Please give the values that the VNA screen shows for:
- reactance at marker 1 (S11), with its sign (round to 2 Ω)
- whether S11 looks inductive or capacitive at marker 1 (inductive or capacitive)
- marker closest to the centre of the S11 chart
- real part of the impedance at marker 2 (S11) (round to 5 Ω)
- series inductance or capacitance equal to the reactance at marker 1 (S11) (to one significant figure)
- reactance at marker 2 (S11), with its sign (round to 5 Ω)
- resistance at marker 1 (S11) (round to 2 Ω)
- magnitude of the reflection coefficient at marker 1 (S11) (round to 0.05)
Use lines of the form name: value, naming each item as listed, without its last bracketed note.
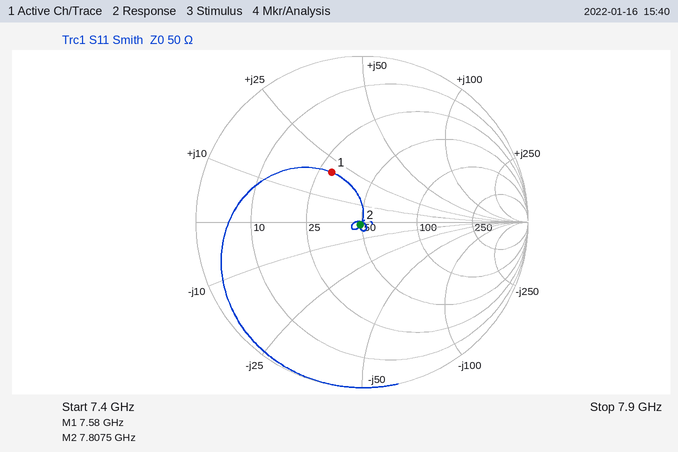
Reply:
reactance at marker 1 (S11), with its sign: +20 Ω
whether S11 looks inductive or capacitive at marker 1: inductive
marker closest to the centre of the S11 chart: marker 2
real part of the impedance at marker 2 (S11): 50 Ω
series inductance or capacitance equal to the reactance at marker 1 (S11): 400 pH
reactance at marker 2 (S11), with its sign: 0 Ω
resistance at marker 1 (S11): 30 Ω
magnitude of the reflection coefficient at marker 1 (S11): 0.35
